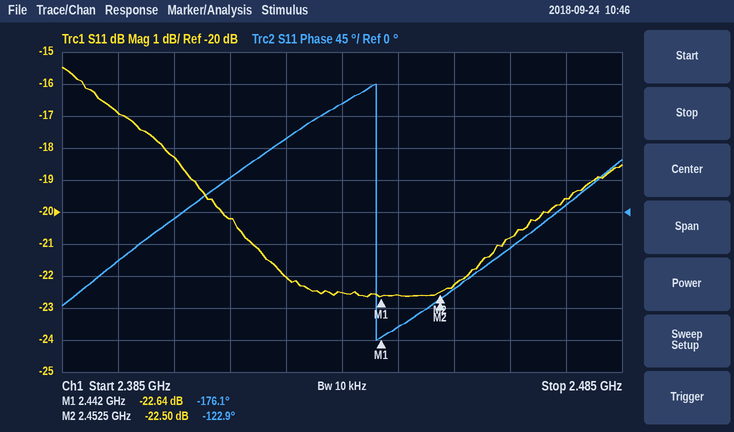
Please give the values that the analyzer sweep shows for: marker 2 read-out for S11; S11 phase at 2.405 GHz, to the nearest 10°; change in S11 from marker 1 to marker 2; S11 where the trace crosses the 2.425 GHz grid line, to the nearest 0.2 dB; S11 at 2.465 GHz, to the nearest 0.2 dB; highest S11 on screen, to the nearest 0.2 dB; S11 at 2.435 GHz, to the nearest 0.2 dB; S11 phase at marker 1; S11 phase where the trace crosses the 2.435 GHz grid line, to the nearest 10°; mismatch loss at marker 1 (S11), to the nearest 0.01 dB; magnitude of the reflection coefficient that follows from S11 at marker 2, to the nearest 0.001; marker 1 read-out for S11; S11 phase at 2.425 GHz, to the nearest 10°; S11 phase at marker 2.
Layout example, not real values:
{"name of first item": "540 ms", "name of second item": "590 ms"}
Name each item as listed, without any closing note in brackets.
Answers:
{"marker 2 read-out for S11": "-22.50 dB", "S11 phase at 2.405 GHz, to the nearest 10°": "-10°", "change in S11 from marker 1 to marker 2": "0.14 dB", "S11 where the trace crosses the 2.425 GHz grid line, to the nearest 0.2 dB": "-22.0 dB", "S11 at 2.465 GHz, to the nearest 0.2 dB": "-20.8 dB", "highest S11 on screen, to the nearest 0.2 dB": "-15.4 dB", "S11 at 2.435 GHz, to the nearest 0.2 dB": "-22.6 dB", "S11 phase at marker 1": "-176.1°", "S11 phase where the trace crosses the 2.435 GHz grid line, to the nearest 10°": "150°", "mismatch loss at marker 1 (S11), to the nearest 0.01 dB": "0.02 dB", "magnitude of the reflection coefficient that follows from S11 at marker 2, to the nearest 0.001": "0.075", "marker 1 read-out for S11": "-22.64 dB", "S11 phase at 2.425 GHz, to the nearest 10°": "100°", "S11 phase at marker 2": "-122.9°"}
